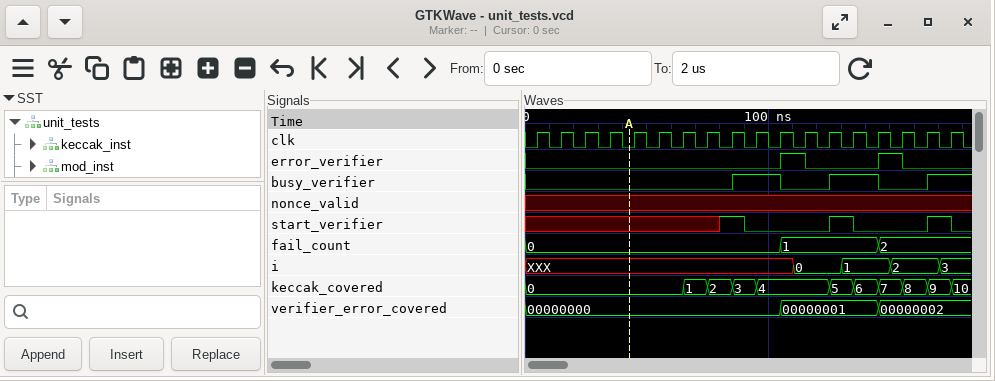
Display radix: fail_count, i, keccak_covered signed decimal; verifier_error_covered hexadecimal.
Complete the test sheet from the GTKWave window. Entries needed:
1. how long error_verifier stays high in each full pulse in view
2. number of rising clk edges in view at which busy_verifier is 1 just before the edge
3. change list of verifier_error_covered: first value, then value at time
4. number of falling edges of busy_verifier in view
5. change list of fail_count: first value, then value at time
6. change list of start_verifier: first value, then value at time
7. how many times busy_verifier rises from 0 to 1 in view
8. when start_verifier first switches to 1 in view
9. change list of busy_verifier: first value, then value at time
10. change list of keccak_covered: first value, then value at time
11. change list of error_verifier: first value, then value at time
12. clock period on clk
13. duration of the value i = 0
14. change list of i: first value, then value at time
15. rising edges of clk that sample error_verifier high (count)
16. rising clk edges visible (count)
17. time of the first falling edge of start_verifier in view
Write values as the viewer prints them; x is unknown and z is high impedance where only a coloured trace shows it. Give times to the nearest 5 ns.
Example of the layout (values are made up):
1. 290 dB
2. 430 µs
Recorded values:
1. 10 ns, 10 ns
2. 5
3. 00000000, 00000001 at 105 ns, 00000002 at 145 ns
4. 2
5. 0, 1 at 105 ns, 2 at 145 ns
6. x, 1 at 80 ns, 0 at 90 ns, 1 at 125 ns, 0 at 135 ns, 1 at 165 ns, 0 at 175 ns
7. 3
8. 80 ns
9. 0, 1 at 85 ns, 0 at 105 ns, 1 at 125 ns, 0 at 145 ns, 1 at 165 ns
10. 0, 1 at 65 ns, 2 at 75 ns, 3 at 85 ns, 4 at 95 ns, 5 at 125 ns, 6 at 135 ns, 7 at 145 ns, 8 at 155 ns, 9 at 165 ns, 10 at 175 ns
11. 0, 1 at 105 ns, 0 at 115 ns, 1 at 145 ns, 0 at 155 ns
12. 10 ns
13. 20 ns
14. XXX, 0 at 110 ns, 1 at 130 ns, 2 at 150 ns, 3 at 170 ns
15. 2
16. 18
17. 90 ns
